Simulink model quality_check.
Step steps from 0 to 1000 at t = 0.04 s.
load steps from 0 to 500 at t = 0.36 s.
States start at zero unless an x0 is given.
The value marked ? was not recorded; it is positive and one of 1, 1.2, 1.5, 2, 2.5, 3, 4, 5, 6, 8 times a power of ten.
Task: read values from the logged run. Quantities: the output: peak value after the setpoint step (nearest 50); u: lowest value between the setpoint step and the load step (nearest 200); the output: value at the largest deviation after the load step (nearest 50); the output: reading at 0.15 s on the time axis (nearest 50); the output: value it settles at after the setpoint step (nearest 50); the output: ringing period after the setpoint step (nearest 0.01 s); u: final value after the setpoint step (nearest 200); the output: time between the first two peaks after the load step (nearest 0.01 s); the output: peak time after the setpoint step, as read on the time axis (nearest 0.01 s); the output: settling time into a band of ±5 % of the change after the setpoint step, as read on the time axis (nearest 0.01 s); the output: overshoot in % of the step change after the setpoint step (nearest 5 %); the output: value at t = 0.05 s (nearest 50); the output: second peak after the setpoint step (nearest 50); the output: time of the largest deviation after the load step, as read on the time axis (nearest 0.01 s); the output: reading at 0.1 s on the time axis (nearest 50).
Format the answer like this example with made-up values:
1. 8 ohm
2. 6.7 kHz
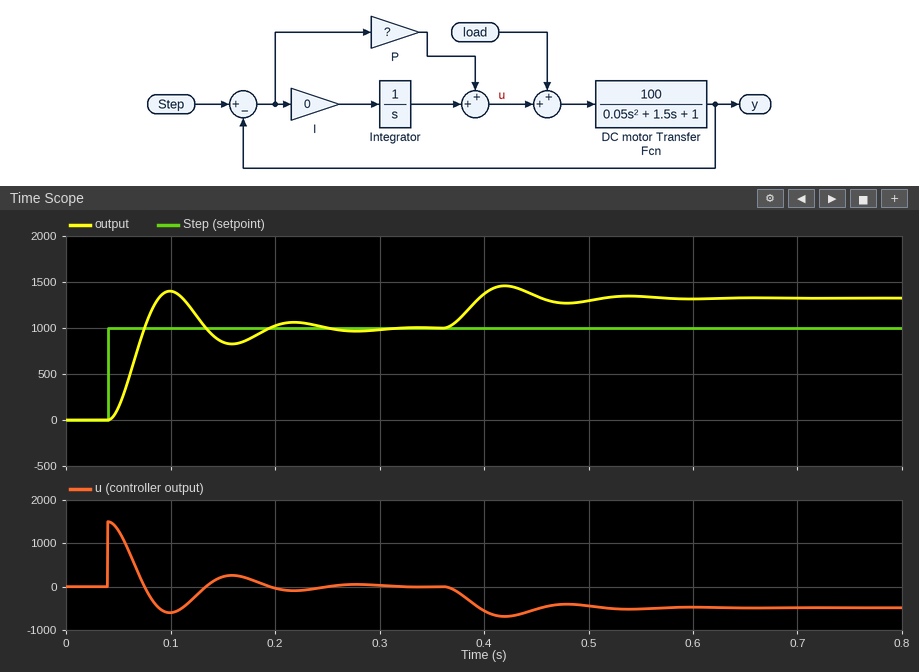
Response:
1. 1400
2. -600
3. 1450
4. 850
5. 1000
6. 0.12 s
7. 0
8. 0.12 s
9. 0.10 s
10. 0.23 s
11. 40 %
12. 150
13. 1050
14. 0.42 s
15. 1400
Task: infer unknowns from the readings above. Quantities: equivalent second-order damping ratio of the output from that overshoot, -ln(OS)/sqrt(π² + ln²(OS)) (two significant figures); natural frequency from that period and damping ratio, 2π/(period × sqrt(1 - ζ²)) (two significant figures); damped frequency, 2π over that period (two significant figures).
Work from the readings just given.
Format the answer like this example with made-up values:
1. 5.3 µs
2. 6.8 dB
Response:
1. 0.28
2. 55 rad/s
3. 52 rad/s
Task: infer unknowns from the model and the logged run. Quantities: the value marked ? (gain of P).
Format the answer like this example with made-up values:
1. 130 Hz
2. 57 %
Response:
1. 1.5
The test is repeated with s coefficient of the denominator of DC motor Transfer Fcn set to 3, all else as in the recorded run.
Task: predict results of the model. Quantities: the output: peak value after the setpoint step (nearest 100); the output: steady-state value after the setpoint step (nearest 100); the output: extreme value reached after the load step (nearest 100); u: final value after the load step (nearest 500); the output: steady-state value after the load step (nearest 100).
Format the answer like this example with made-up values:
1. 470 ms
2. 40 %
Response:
1. 1100
2. 1000
3. 1400
4. -500
5. 1300
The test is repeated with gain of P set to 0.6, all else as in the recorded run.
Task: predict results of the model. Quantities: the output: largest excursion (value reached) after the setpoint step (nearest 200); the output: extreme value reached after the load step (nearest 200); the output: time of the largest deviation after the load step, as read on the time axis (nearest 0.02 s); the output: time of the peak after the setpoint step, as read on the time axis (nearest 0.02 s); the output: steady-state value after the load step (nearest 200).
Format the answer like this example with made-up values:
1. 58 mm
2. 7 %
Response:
1. 1200
2. 2000
3. 0.46 s
4. 0.14 s
5. 1800
